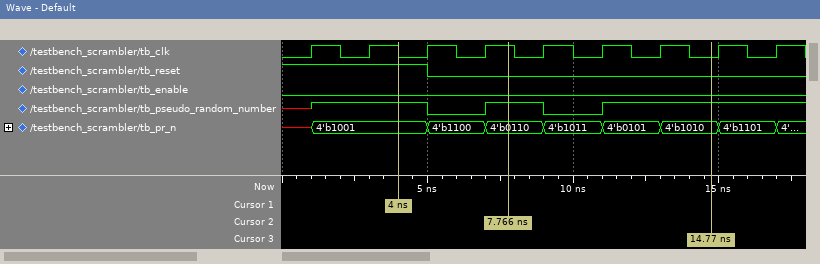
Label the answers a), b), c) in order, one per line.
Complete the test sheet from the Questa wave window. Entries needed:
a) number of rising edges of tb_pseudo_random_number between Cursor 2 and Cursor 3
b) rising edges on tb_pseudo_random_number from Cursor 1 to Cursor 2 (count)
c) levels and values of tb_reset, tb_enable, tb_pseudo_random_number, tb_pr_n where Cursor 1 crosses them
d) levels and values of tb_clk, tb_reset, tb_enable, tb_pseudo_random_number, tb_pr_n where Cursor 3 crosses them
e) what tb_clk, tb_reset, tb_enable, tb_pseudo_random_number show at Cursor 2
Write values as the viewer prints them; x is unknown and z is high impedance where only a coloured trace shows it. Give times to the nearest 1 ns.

a) 1
b) 1
c) tb_reset=1, tb_enable=0, tb_pseudo_random_number=1, tb_pr_n=4'b1001
d) tb_clk=0, tb_reset=0, tb_enable=0, tb_pseudo_random_number=1, tb_pr_n=4'b1010
e) tb_clk=1, tb_reset=0, tb_enable=0, tb_pseudo_random_number=1
